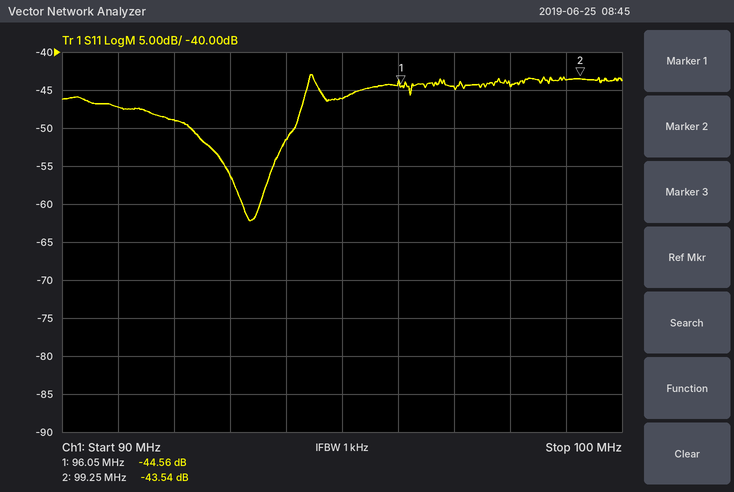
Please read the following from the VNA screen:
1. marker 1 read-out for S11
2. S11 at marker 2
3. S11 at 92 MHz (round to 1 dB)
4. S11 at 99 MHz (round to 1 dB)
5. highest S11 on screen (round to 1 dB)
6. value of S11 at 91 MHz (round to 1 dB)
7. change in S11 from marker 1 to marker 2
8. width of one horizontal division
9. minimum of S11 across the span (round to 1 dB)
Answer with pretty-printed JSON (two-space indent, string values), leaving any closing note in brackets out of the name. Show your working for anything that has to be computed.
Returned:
{
  "marker 1 read-out for S11": "-44.56 dB",
  "S11 at marker 2": "-43.54 dB",
  "S11 at 92 MHz": "-49 dB",
  "S11 at 99 MHz": "-44 dB",
  "highest S11 on screen": "-43 dB",
  "value of S11 at 91 MHz": "-47 dB",
  "change in S11 from marker 1 to marker 2": "-43.54 − (-44.56) = 1.02 dB",
  "width of one horizontal division": "1 MHz",
  "minimum of S11 across the span": "-62 dB"
}
